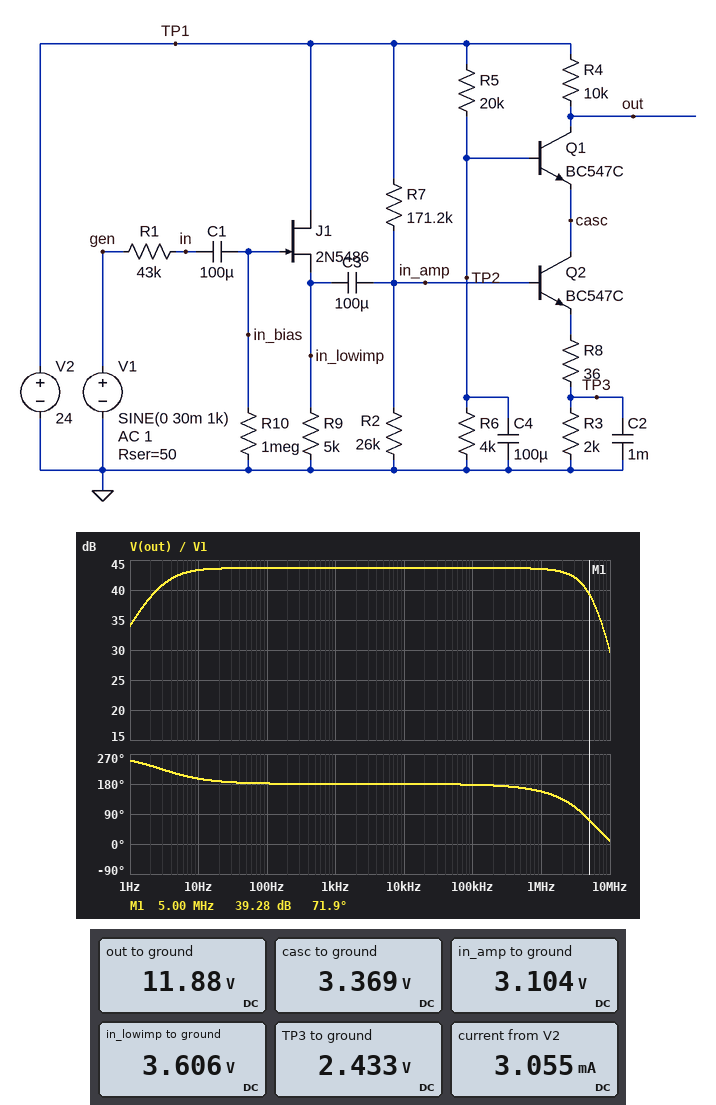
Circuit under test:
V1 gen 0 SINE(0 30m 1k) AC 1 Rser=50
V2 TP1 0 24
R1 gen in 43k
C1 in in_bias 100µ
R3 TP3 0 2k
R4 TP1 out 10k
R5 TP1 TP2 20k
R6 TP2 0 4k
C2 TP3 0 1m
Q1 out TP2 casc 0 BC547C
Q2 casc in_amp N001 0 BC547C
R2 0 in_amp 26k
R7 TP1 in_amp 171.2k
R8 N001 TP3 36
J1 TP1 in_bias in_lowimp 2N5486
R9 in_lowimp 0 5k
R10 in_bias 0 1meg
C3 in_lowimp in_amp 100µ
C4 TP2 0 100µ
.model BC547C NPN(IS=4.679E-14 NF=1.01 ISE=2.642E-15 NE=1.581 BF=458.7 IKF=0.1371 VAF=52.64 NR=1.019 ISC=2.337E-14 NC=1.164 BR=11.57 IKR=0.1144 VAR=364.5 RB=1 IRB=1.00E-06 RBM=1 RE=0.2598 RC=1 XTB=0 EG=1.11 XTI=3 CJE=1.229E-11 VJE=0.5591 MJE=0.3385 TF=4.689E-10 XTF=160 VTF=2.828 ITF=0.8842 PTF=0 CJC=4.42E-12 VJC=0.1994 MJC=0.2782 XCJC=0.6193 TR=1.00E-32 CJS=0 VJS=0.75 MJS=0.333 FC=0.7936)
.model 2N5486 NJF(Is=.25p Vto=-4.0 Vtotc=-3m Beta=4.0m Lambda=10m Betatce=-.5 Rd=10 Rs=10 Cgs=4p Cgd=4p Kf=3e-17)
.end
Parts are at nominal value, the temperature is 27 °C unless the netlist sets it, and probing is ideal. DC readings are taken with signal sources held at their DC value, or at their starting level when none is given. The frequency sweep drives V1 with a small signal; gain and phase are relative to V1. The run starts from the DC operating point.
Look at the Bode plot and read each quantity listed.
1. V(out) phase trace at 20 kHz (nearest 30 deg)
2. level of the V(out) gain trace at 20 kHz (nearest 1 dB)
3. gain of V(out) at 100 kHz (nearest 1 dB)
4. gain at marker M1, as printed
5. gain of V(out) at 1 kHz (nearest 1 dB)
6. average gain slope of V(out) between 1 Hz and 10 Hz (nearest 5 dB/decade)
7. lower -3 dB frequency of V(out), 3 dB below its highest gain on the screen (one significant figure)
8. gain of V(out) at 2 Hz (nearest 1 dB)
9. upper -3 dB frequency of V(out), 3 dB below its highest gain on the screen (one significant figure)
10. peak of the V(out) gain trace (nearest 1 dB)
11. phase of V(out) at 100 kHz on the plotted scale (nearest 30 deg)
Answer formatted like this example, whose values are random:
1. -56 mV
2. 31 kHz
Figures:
1. 180 deg
2. 44 dB
3. 44 dB
4. 39.28 dB
5. 44 dB
6. 10 dB/decade
7. 3 Hz
8. 39 dB
9. 4 MHz
10. 44 dB
11. 180 deg
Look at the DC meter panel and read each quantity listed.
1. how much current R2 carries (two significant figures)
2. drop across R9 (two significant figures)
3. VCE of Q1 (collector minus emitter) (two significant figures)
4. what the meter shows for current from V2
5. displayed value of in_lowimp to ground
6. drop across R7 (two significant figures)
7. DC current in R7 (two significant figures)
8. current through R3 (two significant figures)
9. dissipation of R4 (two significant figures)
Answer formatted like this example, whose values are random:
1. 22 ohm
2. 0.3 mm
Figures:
1. 120 µA
2. 3.6 V
3. 8.5 V
4. 3.055 mA
5. 3.606 V
6. 21 V
7. 120 µA
8. 1.2 mA
9. 15 mW
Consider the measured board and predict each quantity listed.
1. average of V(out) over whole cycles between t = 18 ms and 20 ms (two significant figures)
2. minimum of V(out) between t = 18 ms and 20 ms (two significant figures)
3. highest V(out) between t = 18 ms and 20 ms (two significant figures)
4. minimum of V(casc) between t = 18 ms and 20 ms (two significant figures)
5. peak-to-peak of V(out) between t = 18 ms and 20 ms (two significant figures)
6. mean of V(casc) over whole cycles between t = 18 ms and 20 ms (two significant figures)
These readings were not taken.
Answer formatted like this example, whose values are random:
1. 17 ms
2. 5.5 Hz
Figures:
1. 12 V
2. 7.1 V
3. 16 V
4. 3.4 V
5. 9.1 V
6. 3.4 V
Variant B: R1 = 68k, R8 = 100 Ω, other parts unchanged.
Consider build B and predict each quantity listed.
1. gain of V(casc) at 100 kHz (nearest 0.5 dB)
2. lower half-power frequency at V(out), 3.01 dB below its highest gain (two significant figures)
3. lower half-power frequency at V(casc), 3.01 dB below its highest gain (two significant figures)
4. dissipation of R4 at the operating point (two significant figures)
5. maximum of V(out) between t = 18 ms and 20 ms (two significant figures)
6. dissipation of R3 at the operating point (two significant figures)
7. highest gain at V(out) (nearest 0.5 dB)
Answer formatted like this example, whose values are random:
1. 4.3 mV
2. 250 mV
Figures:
1. -14.5 dB
2. 1.4 Hz
3. 1.3 Hz
4. 14 mW
5. 14 V
6. 2.8 mW
7. 37.0 dB
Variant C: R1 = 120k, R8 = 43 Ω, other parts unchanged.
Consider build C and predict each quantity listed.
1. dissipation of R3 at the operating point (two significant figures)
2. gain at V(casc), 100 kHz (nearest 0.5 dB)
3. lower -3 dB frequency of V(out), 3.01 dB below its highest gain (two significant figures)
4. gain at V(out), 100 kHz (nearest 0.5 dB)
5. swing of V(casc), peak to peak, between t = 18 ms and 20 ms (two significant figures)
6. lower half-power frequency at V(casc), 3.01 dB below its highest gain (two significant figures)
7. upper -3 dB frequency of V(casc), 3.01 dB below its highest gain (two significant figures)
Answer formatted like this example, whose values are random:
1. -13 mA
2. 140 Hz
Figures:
1. 2.9 mW
2. -9.5 dB
3. 2.6 Hz
4. 42.0 dB
5. 20 mV
6. 2.5 Hz
7. 1.7 MHz
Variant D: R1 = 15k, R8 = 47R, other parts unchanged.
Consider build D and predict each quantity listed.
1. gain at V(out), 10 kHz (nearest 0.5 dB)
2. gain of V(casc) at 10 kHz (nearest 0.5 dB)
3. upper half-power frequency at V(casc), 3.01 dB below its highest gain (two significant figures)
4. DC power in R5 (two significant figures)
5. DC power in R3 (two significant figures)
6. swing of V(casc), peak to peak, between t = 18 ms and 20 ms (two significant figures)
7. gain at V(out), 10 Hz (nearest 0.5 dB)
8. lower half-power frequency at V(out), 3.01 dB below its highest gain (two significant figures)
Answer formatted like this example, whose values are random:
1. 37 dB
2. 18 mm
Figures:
1. 42.5 dB
2. -9.0 dB
3. 10 MHz
4. 20 mW
5. 2.9 mW
6. 21 mV
7. 42.0 dB
8. 2.4 Hz
